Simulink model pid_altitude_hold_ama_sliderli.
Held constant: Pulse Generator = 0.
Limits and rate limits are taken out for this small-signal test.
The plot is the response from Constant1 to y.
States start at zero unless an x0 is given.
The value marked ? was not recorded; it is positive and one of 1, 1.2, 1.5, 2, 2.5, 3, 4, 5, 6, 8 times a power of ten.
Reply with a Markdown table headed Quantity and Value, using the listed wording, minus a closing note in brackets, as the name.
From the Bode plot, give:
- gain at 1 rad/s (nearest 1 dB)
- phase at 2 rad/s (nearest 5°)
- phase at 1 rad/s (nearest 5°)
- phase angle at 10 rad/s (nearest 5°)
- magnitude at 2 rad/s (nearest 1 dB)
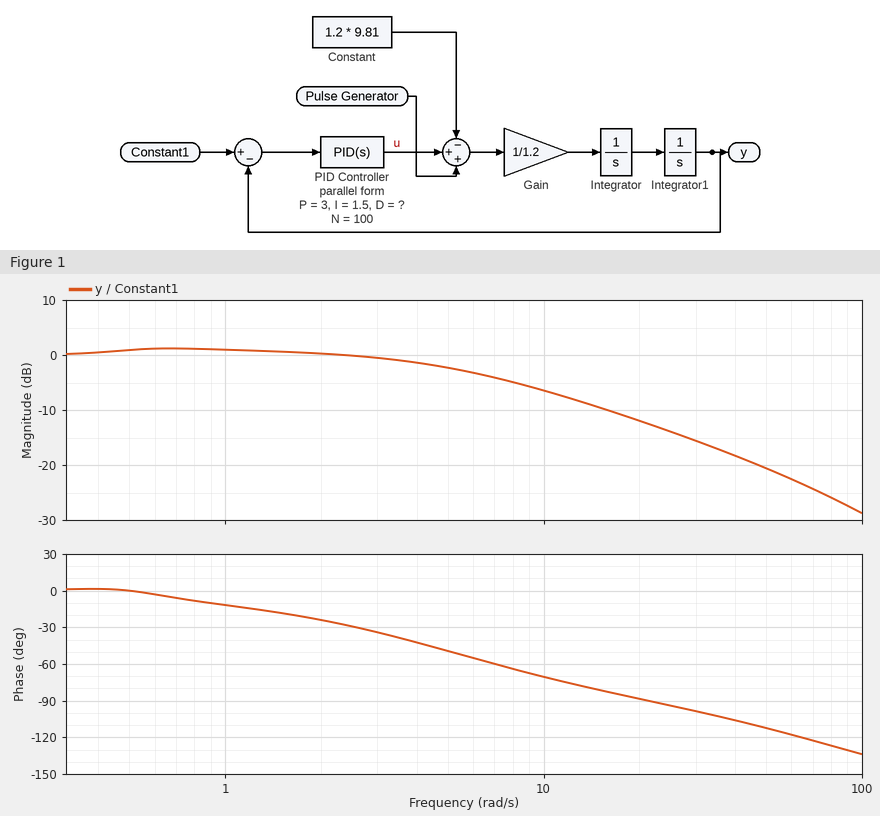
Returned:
| Quantity | Value |
|---|---|
| gain at 1 rad/s | 1 dB |
| phase at 2 rad/s | -25° |
| phase at 1 rad/s | -10° |
| phase angle at 10 rad/s | -70° |
| magnitude at 2 rad/s | 0 dB |
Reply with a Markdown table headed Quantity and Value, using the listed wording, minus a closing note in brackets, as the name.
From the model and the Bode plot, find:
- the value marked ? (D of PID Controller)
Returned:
| Quantity | Value |
|---|---|
| the value marked ? | 6 |
